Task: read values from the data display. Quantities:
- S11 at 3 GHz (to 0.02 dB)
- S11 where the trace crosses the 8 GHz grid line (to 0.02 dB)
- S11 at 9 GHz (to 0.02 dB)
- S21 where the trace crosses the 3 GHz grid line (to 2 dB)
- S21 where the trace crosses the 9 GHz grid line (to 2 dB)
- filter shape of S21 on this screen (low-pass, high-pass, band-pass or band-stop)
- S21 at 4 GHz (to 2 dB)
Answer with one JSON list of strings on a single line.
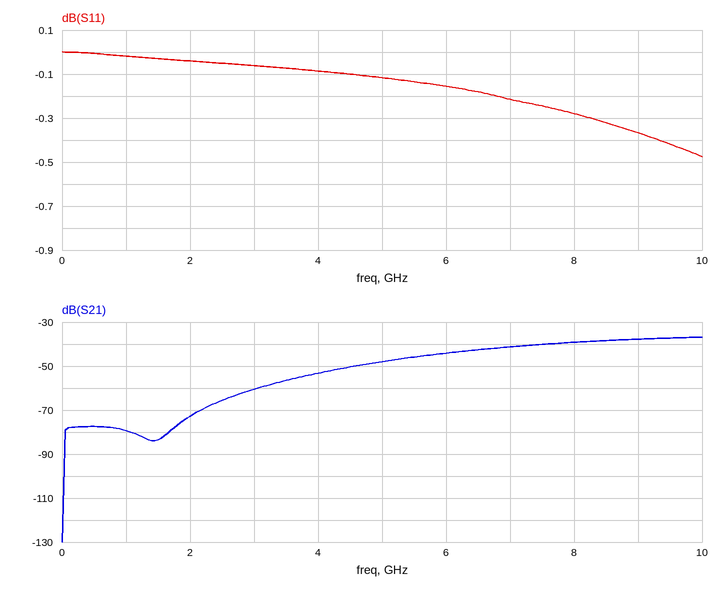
["-0.06 dB", "-0.28 dB", "-0.36 dB", "-60 dB", "-38 dB", "high-pass", "-54 dB"]
